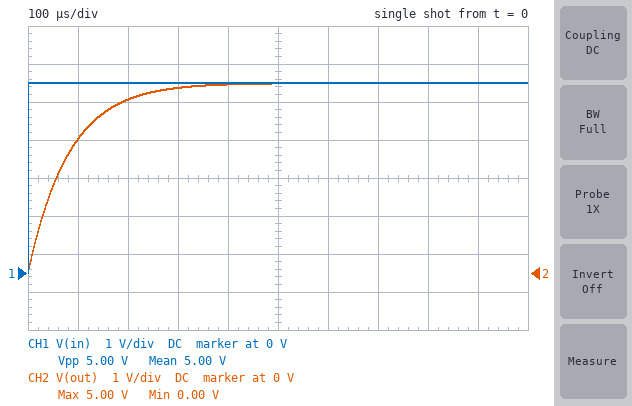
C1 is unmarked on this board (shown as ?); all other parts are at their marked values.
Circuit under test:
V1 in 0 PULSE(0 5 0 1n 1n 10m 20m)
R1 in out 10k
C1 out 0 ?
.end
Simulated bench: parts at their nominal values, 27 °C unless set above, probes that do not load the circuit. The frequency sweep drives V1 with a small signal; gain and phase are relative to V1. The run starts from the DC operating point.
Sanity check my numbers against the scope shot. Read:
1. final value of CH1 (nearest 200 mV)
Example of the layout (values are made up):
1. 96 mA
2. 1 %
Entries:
1. 5.0 V
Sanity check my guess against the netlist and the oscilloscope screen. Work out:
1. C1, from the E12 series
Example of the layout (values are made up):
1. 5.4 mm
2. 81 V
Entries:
1. 8.2 nF
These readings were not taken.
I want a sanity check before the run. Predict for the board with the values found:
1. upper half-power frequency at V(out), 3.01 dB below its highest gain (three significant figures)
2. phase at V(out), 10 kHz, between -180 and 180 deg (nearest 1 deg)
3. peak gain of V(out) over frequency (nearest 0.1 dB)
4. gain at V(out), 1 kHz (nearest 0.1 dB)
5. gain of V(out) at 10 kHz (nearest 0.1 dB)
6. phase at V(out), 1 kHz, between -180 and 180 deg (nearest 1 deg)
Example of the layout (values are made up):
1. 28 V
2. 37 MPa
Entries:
1. 1.94 kHz
2. -79 deg
3. 0 dB
4. -1.0 dB
5. -14.4 dB
6. -27 deg
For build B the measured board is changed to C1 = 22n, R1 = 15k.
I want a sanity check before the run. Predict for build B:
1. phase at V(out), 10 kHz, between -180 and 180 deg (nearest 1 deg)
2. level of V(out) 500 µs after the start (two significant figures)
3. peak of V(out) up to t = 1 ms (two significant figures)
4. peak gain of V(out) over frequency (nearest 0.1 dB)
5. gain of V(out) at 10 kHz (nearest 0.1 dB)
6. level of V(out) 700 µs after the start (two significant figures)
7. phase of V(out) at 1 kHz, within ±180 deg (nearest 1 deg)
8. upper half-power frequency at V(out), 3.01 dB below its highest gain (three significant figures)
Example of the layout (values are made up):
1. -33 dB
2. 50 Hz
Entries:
1. -87 deg
2. 3.9 V
3. 4.8 V
4. 0 dB
5. -26.3 dB
6. 4.4 V
7. -64 deg
8. 482 Hz
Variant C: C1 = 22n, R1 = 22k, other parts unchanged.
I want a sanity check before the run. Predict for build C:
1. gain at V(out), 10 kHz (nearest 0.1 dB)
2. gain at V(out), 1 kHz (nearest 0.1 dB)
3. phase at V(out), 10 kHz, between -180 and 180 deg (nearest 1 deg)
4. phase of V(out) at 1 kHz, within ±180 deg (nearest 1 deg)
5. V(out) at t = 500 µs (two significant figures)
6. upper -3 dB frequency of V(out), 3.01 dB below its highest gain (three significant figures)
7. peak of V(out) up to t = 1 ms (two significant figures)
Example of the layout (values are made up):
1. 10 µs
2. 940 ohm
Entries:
1. -29.7 dB
2. -10.1 dB
3. -88 deg
4. -72 deg
5. 3.2 V
6. 329 Hz
7. 4.4 V
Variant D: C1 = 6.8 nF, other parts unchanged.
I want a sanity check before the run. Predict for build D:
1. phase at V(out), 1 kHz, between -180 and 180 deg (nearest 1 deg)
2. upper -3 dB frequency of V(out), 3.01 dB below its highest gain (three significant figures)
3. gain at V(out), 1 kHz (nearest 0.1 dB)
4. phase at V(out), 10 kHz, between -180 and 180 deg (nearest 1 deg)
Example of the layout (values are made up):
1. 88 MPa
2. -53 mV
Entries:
1. -23 deg
2. 2.34 kHz
3. -0.7 dB
4. -77 deg
